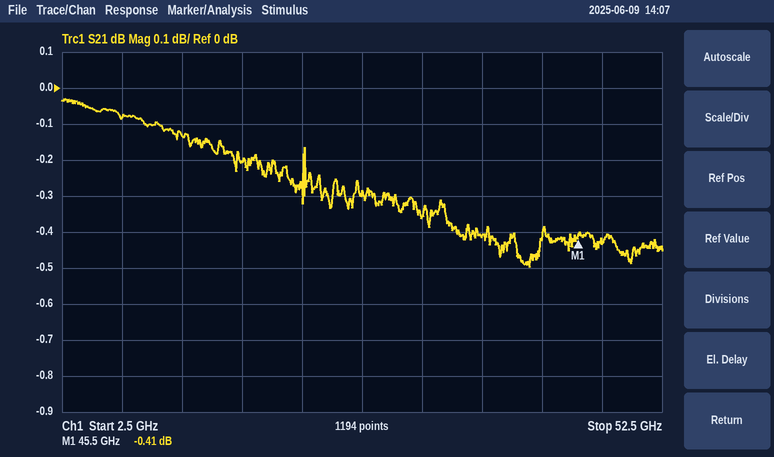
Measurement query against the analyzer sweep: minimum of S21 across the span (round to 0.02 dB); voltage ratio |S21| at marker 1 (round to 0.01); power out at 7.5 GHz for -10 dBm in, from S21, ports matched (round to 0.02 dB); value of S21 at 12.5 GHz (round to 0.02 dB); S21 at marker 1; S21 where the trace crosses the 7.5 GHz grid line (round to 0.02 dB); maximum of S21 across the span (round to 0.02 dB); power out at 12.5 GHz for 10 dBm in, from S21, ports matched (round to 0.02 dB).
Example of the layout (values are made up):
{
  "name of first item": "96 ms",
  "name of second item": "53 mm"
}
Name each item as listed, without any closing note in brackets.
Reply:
{
  "minimum of S21 across the span": "-0.50 dB",
  "voltage ratio |S21| at marker 1": "0.95",
  "power out at 7.5 GHz for -10 dBm in, from S21, ports matched": "-10.08 dBm",
  "value of S21 at 12.5 GHz": "-0.14 dB",
  "S21 at marker 1": "-0.41 dB",
  "S21 where the trace crosses the 7.5 GHz grid line": "-0.08 dB",
  "maximum of S21 across the span": "-0.02 dB",
  "power out at 12.5 GHz for 10 dBm in, from S21, ports matched": "9.86 dBm"
}
